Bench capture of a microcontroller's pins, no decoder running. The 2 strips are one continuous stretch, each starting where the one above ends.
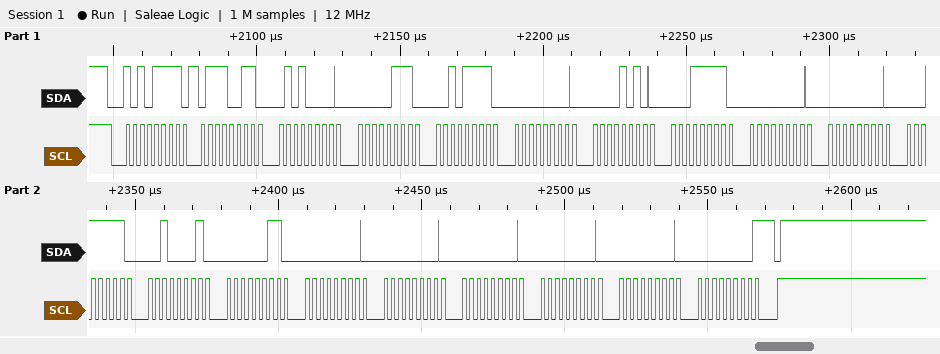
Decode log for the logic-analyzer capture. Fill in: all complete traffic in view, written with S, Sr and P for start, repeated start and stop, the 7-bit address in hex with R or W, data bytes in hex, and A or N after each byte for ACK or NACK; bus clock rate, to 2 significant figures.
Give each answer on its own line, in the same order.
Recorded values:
S 57R A 73 A 50 A 07 A 2F A 00 A 0A A 1F A 00 A 00 A 1F A 21 A 03 A 00 A 00 A 00 A 00 A 00 A 00 N P
400 kHz
